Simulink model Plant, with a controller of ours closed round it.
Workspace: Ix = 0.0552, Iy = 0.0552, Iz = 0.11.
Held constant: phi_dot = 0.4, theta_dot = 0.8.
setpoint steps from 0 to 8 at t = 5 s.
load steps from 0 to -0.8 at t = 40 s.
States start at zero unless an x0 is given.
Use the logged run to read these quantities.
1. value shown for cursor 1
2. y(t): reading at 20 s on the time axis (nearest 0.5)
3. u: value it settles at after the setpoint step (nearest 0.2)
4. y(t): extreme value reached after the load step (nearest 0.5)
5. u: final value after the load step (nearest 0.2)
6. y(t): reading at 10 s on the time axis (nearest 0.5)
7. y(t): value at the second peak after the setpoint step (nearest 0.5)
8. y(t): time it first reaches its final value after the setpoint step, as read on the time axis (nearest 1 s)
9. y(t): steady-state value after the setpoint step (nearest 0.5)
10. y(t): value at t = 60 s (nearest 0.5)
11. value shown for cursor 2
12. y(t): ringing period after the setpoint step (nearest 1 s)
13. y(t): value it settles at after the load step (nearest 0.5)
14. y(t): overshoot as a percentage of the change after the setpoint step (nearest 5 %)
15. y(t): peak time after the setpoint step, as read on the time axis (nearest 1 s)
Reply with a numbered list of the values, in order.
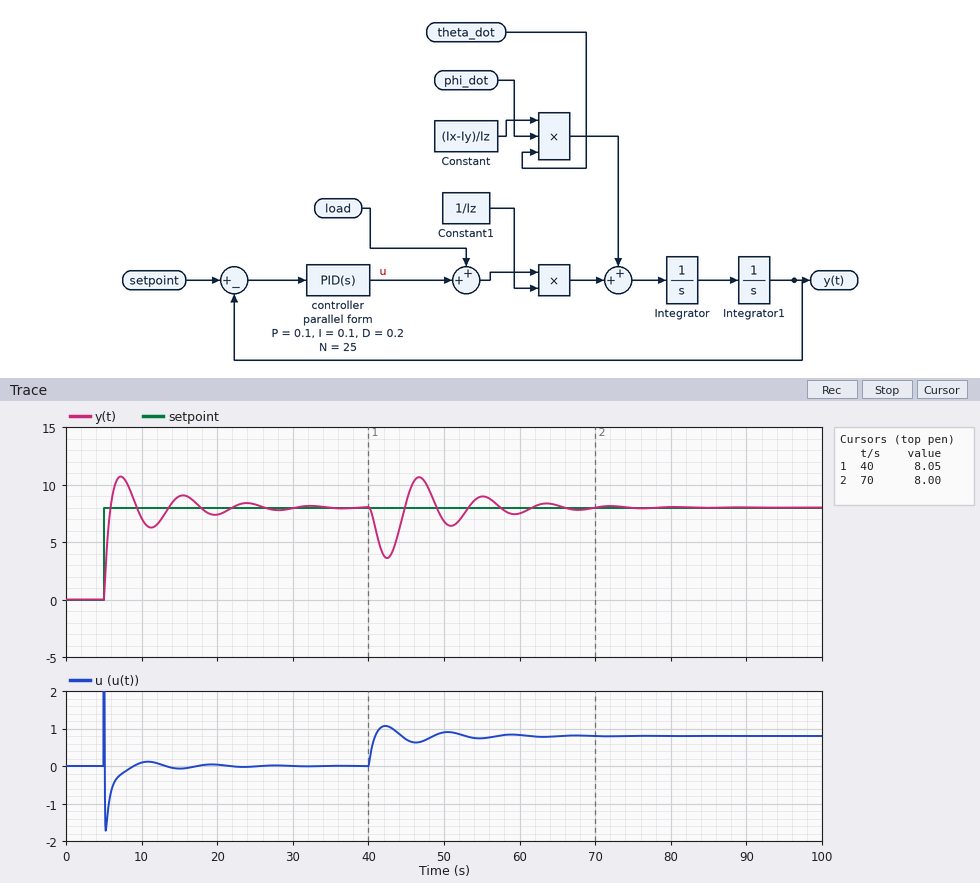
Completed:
1. 8.05
2. 7.5
3. 0.0
4. 3.5
5. 0.8
6. 7.0
7. 9.0
8. 6 s
9. 8.0
10. 7.5
11. 8.00
12. 8 s
13. 8.0
14. 35 %
15. 7 s
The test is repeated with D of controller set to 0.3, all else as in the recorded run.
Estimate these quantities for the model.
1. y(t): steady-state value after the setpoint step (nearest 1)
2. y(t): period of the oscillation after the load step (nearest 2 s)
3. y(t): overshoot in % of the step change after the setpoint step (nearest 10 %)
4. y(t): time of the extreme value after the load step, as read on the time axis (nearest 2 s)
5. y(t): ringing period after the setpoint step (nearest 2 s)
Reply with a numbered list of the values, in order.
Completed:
1. 8
2. 10 s
3. 20 %
4. 42 s
5. 10 s
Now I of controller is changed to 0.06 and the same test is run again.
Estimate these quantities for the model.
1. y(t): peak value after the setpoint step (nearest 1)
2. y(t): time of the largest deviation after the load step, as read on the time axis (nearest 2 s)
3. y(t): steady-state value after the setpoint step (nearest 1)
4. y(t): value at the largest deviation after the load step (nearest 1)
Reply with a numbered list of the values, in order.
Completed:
1. 10
2. 42 s
3. 8
4. 3
